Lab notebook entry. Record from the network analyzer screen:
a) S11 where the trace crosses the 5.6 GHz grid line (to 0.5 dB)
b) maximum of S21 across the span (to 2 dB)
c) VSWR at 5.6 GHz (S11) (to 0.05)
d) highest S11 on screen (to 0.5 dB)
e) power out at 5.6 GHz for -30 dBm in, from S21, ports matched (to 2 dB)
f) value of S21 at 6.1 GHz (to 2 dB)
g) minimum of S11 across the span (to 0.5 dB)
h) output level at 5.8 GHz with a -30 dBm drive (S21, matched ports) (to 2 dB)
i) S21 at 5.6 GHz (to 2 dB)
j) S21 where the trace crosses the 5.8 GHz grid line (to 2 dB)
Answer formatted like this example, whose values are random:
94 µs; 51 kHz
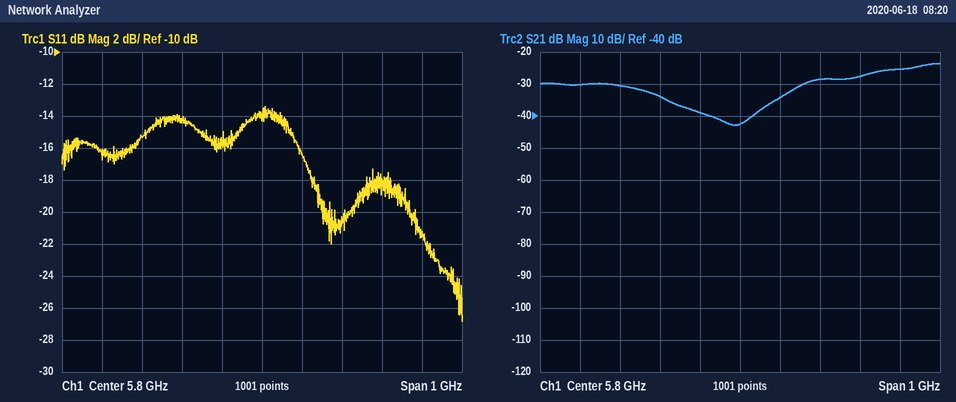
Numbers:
-14.0 dB; -24 dB; 1.50; -13.5 dB; -64 dBm; -28 dB; -27.0 dB; -72 dBm; -34 dB; -42 dB
